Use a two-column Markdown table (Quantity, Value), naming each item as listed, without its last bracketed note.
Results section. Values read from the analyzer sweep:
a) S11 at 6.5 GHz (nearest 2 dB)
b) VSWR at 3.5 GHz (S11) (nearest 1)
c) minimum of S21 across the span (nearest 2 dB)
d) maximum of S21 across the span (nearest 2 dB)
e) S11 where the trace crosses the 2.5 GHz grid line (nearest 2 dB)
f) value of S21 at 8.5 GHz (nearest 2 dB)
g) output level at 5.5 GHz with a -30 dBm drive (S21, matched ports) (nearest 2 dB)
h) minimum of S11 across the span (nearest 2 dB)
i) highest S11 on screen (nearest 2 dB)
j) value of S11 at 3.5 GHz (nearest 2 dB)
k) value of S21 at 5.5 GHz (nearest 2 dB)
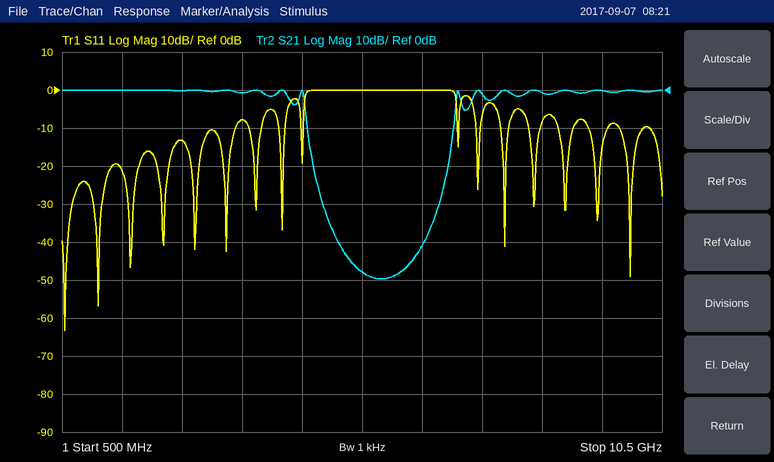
| Quantity | Value |
|---|---|
| S11 at 6.5 GHz | 0 dB |
| VSWR at 3.5 GHz (S11) | 2 |
| minimum of S21 across the span | -50 dB |
| maximum of S21 across the span | 0 dB |
| S11 where the trace crosses the 2.5 GHz grid line | -14 dB |
| value of S21 at 8.5 GHz | 0 dB |
| output level at 5.5 GHz with a -30 dBm drive (S21, matched ports) | -78 dBm |
| minimum of S11 across the span | -64 dB |
| highest S11 on screen | 0 dB |
| value of S11 at 3.5 GHz | -8 dB |
| value of S21 at 5.5 GHz | -48 dB |
